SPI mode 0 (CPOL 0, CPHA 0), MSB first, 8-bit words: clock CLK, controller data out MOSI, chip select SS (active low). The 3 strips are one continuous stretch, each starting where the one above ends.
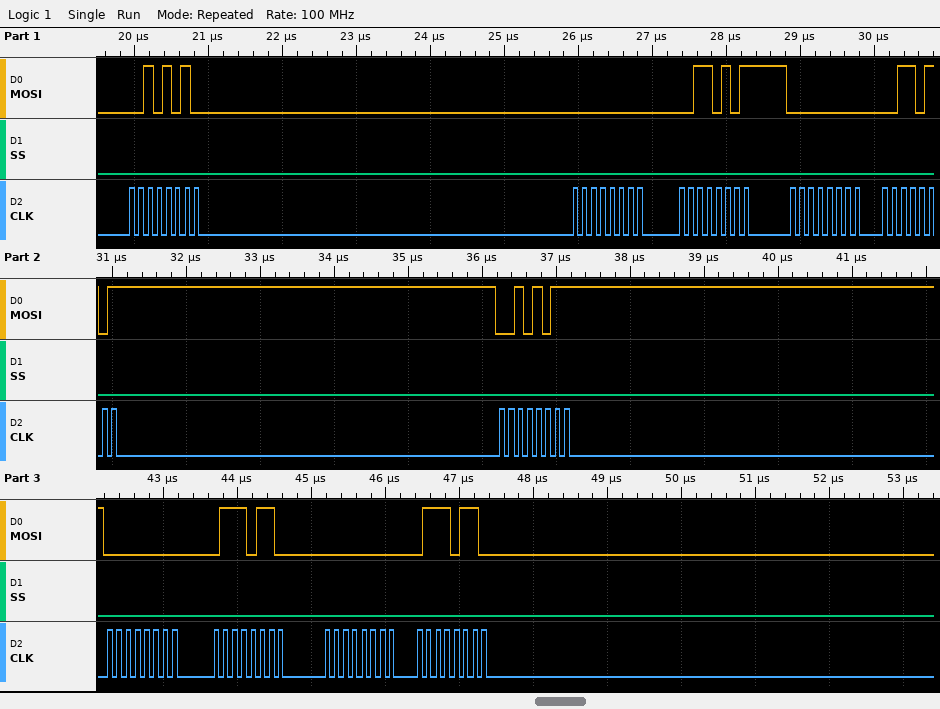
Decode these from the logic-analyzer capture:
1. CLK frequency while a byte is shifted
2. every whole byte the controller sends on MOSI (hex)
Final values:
8 MHz
2A 00 35 00 35 2B 00 76 00 76
